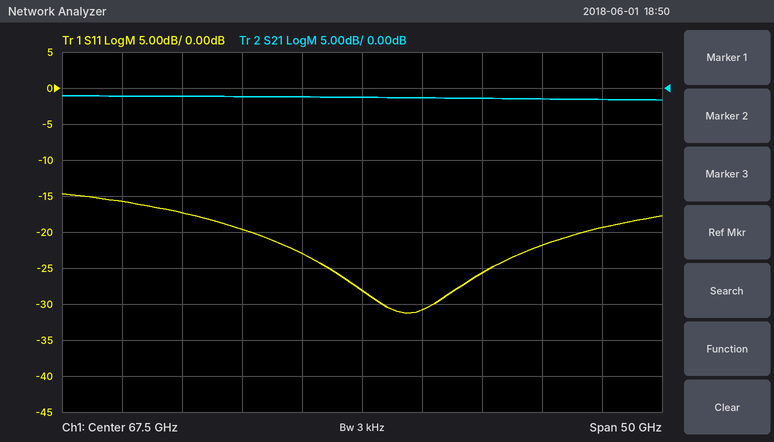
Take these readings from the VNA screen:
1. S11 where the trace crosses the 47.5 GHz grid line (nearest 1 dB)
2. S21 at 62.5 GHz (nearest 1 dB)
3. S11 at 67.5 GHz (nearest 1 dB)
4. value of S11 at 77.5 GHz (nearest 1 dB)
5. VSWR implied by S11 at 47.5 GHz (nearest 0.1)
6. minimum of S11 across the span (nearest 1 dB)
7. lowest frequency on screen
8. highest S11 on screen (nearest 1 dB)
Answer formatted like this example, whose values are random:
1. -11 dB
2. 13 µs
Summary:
1. -16 dB
2. -1 dB
3. -28 dB
4. -26 dB
5. 1.4
6. -31 dB
7. 42.5 GHz
8. -15 dB
